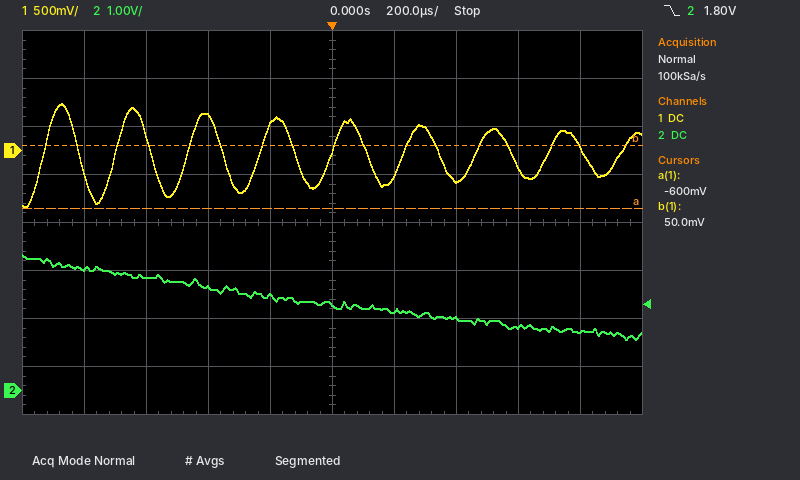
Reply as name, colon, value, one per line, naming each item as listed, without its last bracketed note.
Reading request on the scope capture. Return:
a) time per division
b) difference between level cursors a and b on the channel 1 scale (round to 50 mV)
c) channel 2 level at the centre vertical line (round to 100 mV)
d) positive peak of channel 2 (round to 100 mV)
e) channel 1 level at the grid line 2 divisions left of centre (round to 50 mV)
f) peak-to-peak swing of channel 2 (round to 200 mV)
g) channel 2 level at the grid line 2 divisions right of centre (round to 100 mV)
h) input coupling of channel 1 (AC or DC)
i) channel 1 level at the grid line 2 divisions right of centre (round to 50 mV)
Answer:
time per division: 200 µs
difference between level cursors a and b on the channel 1 scale: 650 mV
channel 2 level at the centre vertical line: 1.8 V
positive peak of channel 2: 2.8 V
channel 1 level at the grid line 2 divisions left of centre: 350 mV
peak-to-peak swing of channel 2: 1.8 V
channel 2 level at the grid line 2 divisions right of centre: 1.5 V
input coupling of channel 1: DC
channel 1 level at the grid line 2 divisions right of centre: -300 mV
